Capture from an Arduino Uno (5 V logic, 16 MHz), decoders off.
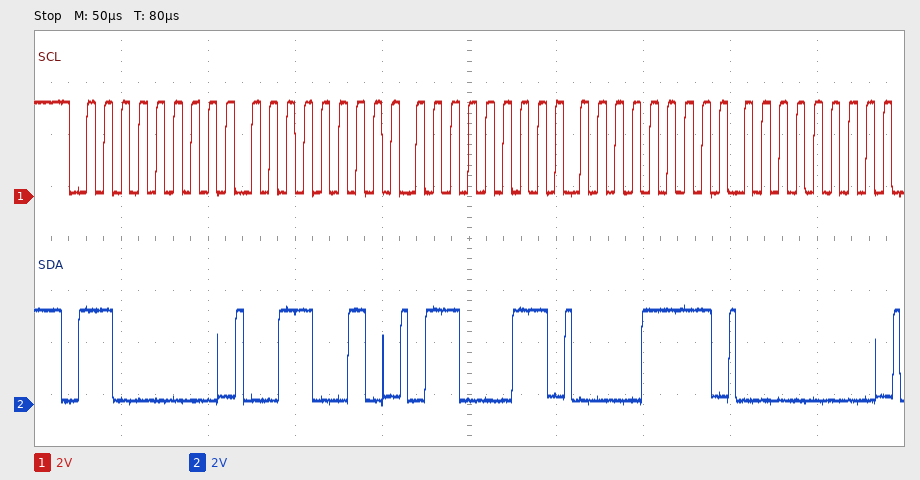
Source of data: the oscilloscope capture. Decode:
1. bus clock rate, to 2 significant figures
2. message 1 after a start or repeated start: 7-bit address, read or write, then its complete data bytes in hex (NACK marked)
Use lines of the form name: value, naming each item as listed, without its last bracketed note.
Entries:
bus clock rate, to 2 significant figures: 100 kHz
message 1 after a start or repeated start: 7-bit address, read or write, then its complete data bytes in hex: 0x60 write: 32 63 0F 00
